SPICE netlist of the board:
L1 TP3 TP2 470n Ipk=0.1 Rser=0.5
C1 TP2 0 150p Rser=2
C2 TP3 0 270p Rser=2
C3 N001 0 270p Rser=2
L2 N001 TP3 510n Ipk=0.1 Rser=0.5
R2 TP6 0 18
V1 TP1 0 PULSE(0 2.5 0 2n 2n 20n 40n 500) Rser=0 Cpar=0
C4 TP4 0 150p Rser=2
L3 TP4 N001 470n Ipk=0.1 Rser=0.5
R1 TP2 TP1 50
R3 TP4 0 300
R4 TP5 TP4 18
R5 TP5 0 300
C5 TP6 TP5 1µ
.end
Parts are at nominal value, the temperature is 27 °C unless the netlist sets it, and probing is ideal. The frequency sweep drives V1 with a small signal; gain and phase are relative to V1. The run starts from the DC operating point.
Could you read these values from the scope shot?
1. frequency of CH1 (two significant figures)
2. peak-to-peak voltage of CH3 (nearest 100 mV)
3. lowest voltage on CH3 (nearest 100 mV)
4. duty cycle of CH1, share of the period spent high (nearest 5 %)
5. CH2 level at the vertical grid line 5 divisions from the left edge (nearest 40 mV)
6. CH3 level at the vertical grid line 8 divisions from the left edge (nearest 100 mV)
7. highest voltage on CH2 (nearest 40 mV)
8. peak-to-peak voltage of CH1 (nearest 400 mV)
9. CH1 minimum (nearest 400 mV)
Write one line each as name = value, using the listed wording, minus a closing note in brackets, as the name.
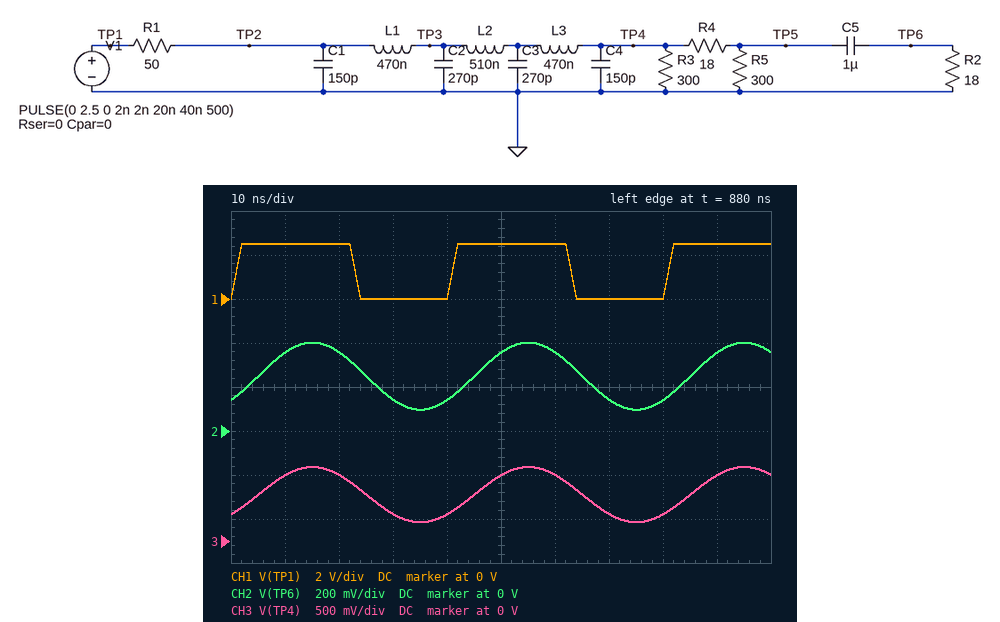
frequency of CH1 = 25 MHz
peak-to-peak voltage of CH3 = 600 mV
lowest voltage on CH3 = 200 mV
duty cycle of CH1, share of the period spent high = 55 %
CH2 level at the vertical grid line 5 divisions from the left edge = 360 mV
CH3 level at the vertical grid line 8 divisions from the left edge = 300 mV
highest voltage on CH2 = 400 mV
peak-to-peak voltage of CH1 = 2.4 V
CH1 minimum = 0 V
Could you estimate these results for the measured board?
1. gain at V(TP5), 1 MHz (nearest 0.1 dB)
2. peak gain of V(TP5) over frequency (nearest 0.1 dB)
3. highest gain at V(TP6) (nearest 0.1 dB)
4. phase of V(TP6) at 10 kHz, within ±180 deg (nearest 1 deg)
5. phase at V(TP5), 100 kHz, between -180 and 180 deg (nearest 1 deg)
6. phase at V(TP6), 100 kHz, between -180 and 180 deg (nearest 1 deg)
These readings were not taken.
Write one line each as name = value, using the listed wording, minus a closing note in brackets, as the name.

gain at V(TP5), 1 MHz = -14.7 dB
peak gain of V(TP5) over frequency = -3.0 dB
highest gain at V(TP6) = -14.6 dB
phase of V(TP6) at 10 kHz, within ±180 deg = 13 deg
phase at V(TP5), 100 kHz, between -180 and 180 deg = -5 deg
phase at V(TP6), 100 kHz, between -180 and 180 deg = 0 deg
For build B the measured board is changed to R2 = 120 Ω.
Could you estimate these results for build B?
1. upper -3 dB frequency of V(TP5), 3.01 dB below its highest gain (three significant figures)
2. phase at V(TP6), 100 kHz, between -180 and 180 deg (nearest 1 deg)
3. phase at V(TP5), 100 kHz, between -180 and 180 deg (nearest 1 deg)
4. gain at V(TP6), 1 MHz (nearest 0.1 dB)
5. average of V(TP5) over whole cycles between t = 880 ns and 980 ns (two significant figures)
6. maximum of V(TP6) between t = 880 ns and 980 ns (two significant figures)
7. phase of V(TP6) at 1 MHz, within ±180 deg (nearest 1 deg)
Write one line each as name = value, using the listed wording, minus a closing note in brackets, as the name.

upper -3 dB frequency of V(TP5), 3.01 dB below its highest gain = 6.72 kHz
phase at V(TP6), 100 kHz, between -180 and 180 deg = -1 deg
phase at V(TP5), 100 kHz, between -180 and 180 deg = -2 deg
gain at V(TP6), 1 MHz = -6.1 dB
average of V(TP5) over whole cycles between t = 880 ns and 980 ns = 680 mV
maximum of V(TP6) between t = 880 ns and 980 ns = 1.1 V
phase of V(TP6) at 1 MHz, within ±180 deg = -13 deg
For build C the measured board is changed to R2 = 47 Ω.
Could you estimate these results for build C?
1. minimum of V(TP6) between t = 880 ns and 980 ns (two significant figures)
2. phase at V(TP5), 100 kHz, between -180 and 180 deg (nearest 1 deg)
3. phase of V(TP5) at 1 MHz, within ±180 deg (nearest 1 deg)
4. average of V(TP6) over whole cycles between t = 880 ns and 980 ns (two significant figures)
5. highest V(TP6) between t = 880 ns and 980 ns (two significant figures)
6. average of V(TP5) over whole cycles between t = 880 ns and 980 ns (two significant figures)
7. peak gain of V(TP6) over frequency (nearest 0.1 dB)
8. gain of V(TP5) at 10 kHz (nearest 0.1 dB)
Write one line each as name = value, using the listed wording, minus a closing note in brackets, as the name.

minimum of V(TP6) between t = 880 ns and 980 ns = 160 mV
phase at V(TP5), 100 kHz, between -180 and 180 deg = -2 deg
phase of V(TP5) at 1 MHz, within ±180 deg = -13 deg
average of V(TP6) over whole cycles between t = 880 ns and 980 ns = 460 mV
highest V(TP6) between t = 880 ns and 980 ns = 760 mV
average of V(TP5) over whole cycles between t = 880 ns and 980 ns = 470 mV
peak gain of V(TP6) over frequency = -9.4 dB
gain of V(TP5) at 10 kHz = -9.1 dB
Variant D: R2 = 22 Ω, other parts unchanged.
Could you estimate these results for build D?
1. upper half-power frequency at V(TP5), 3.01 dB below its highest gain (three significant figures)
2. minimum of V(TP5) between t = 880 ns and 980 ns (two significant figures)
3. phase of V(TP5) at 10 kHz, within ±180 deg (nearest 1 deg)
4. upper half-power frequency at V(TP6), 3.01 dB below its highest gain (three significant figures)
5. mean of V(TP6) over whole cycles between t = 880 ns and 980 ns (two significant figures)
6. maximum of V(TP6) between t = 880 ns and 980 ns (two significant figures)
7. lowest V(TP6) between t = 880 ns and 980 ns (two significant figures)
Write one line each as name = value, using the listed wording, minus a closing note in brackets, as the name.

upper half-power frequency at V(TP5), 3.01 dB below its highest gain = 2.40 kHz
minimum of V(TP5) between t = 880 ns and 980 ns = 120 mV
phase of V(TP5) at 10 kHz, within ±180 deg = -24 deg
upper half-power frequency at V(TP6), 3.01 dB below its highest gain = 22.6 MHz
mean of V(TP6) over whole cycles between t = 880 ns and 980 ns = 290 mV
maximum of V(TP6) between t = 880 ns and 980 ns = 470 mV
lowest V(TP6) between t = 880 ns and 980 ns = 110 mV
